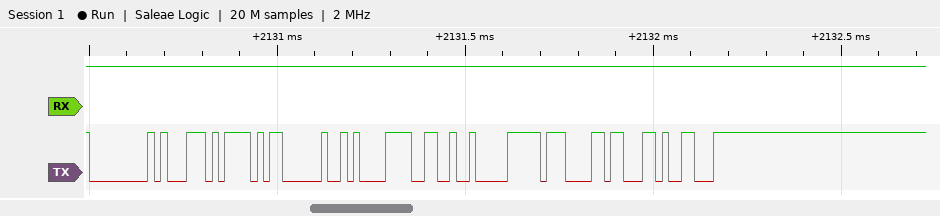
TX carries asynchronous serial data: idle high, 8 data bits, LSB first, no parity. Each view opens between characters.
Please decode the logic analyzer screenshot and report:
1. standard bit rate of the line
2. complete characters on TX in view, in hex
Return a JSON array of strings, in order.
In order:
["57600 baud", "00, 71, AF, 20, E1, 26, F0, 87, 63, C6"]
